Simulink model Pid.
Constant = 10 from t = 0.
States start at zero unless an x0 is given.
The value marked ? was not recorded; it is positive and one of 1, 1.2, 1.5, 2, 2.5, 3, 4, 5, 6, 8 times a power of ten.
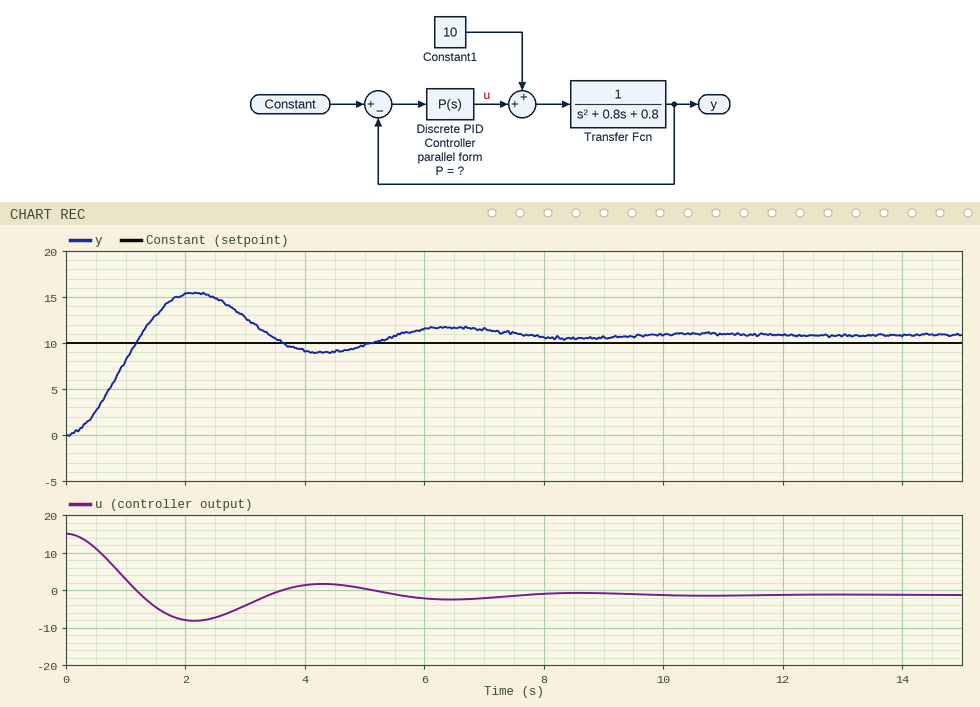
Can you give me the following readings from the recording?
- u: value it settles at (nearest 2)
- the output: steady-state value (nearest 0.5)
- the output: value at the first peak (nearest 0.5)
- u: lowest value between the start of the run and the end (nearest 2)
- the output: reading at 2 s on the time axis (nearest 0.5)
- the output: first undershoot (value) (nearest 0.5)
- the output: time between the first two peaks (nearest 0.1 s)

-2
11.0
15.5
-8
15.5
9.0
4.3 s
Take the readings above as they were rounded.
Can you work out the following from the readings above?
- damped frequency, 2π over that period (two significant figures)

1.5 rad/s
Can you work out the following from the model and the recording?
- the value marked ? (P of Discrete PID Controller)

1.5
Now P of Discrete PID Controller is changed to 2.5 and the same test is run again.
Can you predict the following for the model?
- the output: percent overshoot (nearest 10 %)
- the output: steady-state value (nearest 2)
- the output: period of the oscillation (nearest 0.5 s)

50 %
10
3.5 s
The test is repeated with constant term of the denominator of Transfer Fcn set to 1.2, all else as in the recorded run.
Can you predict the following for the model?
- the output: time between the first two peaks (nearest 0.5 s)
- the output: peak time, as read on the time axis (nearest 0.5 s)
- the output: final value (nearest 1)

4.0 s
2.0 s
9
